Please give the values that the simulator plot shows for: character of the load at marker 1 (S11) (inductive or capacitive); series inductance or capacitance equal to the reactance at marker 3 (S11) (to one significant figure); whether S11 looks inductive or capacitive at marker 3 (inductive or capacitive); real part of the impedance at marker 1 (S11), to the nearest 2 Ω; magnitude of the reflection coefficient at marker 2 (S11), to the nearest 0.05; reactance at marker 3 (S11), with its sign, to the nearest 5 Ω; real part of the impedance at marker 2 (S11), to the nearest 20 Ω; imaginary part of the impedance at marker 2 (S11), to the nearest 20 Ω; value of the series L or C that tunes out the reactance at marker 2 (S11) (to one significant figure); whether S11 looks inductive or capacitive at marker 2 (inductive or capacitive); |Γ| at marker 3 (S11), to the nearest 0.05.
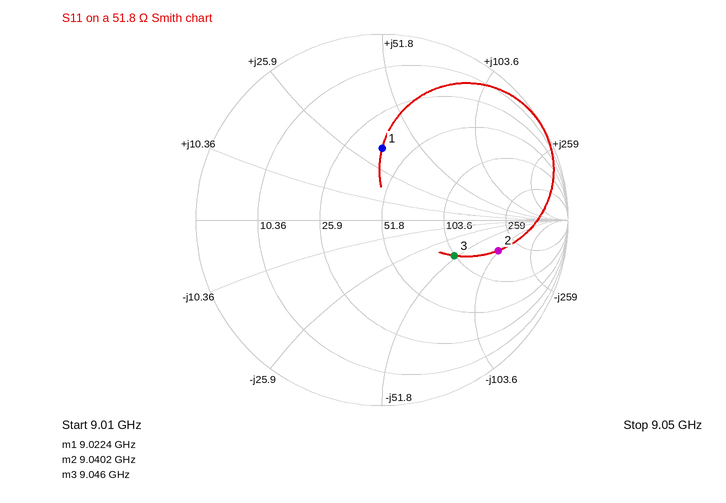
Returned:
inductive
400 fF
capacitive
38 Ω
0.65
-50 Ω
180 Ω
-100 Ω
2 nH
capacitive
0.45
